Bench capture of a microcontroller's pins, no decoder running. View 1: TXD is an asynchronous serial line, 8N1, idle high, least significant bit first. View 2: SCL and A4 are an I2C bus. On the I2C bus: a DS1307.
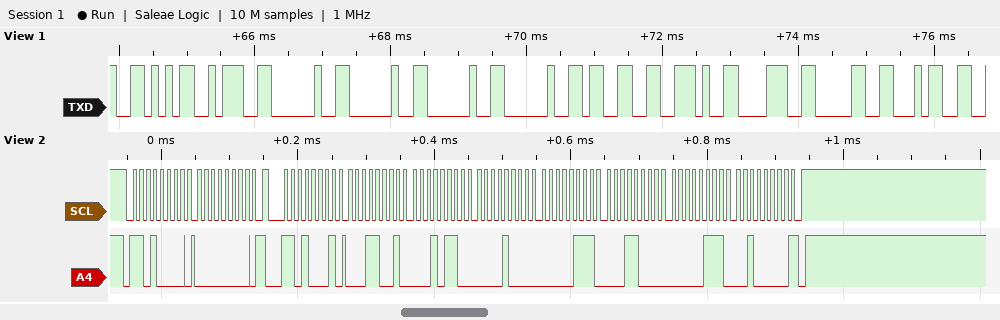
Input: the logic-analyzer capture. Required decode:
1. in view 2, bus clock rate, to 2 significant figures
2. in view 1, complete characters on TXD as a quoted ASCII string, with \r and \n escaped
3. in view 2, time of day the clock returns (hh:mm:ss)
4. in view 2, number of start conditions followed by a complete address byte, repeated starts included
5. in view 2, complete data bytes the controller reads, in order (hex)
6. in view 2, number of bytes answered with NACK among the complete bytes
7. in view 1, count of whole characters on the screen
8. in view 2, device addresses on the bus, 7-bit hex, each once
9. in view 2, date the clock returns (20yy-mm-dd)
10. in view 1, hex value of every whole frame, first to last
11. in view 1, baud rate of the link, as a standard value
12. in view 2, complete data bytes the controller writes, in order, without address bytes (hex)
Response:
100 kHz
"V:    3.804"
08:16:19
2
19 16 08 07 18 07 20
1
11
0x68
2020-07-18
56 3A 20 20 20 20 33 2E 38 30 34
9600 baud
00
